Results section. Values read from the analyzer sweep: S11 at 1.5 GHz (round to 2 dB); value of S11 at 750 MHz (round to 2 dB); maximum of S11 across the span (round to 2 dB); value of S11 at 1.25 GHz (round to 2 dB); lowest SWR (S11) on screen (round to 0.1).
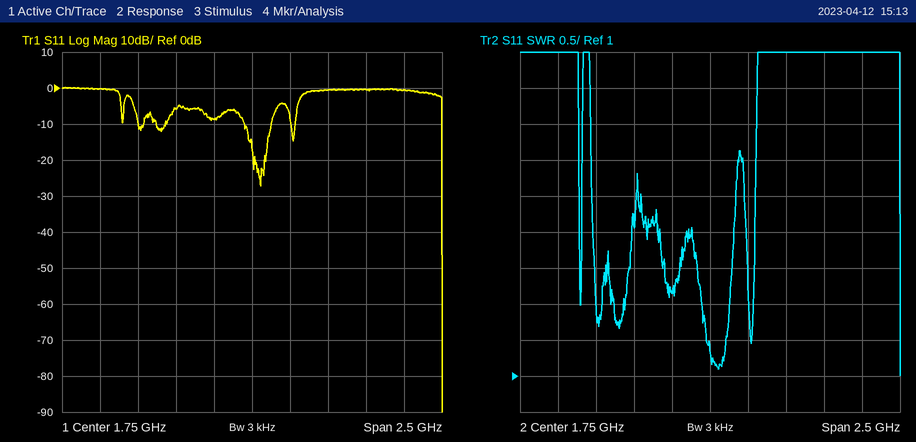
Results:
-8 dB
0 dB
0 dB
-6 dB
1.0
